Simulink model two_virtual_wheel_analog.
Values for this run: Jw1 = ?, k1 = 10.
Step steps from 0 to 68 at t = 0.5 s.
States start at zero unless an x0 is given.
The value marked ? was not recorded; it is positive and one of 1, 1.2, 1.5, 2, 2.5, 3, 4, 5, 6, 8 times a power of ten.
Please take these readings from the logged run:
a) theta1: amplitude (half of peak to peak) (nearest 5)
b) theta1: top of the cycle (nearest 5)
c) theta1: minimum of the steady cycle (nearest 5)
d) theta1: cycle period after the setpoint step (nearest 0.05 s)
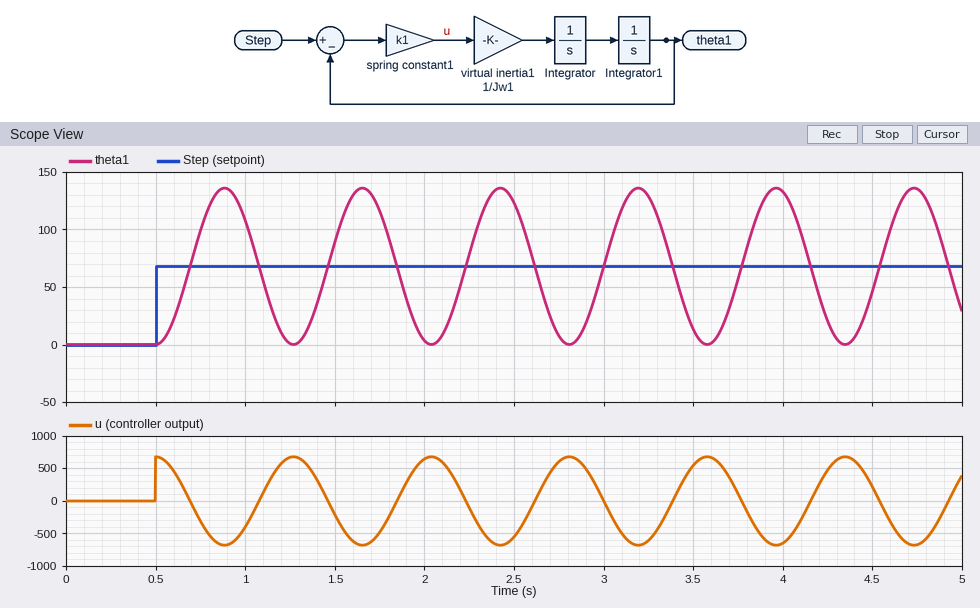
70
135
0
0.75 s
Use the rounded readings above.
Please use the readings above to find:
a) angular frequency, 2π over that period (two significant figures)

8.4 rad/s
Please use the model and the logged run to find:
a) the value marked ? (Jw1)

0.15
